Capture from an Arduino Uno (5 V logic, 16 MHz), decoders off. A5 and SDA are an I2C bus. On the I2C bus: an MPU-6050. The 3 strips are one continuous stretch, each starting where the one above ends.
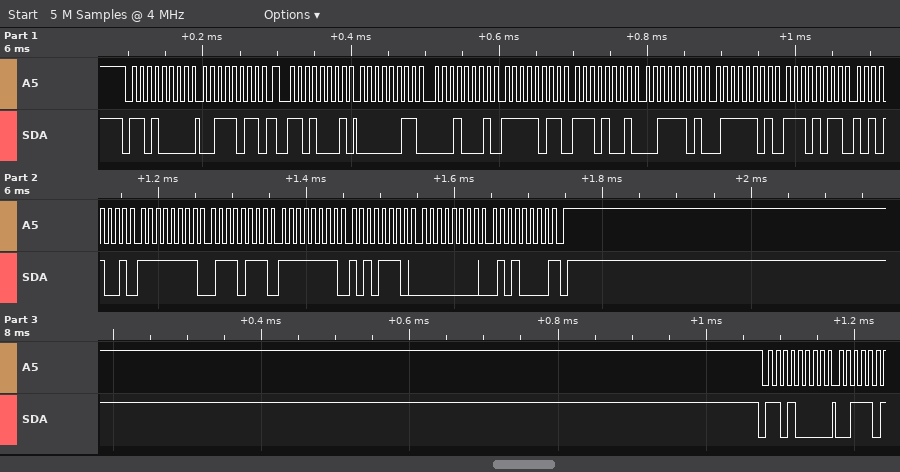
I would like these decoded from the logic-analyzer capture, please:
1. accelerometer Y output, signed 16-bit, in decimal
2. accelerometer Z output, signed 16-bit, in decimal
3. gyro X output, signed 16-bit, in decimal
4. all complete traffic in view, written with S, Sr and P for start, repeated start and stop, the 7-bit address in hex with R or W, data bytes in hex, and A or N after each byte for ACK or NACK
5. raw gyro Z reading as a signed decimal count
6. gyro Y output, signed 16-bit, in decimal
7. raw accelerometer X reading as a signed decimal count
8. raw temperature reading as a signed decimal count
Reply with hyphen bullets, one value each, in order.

- -1047
- 15741
- -137
- S 68W A 3B A Sr 68R A 03 A 11 A FB A E9 A 3D A 7D A EB A A9 A FF A 77 A FF A AE A 00 A 50 N P S 68W A
- 80
- -82
- 785
- -5207
